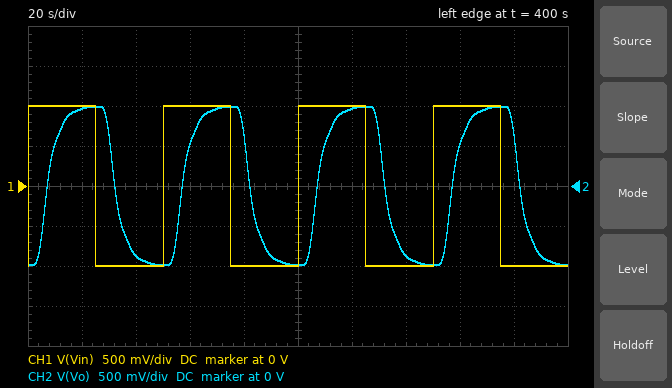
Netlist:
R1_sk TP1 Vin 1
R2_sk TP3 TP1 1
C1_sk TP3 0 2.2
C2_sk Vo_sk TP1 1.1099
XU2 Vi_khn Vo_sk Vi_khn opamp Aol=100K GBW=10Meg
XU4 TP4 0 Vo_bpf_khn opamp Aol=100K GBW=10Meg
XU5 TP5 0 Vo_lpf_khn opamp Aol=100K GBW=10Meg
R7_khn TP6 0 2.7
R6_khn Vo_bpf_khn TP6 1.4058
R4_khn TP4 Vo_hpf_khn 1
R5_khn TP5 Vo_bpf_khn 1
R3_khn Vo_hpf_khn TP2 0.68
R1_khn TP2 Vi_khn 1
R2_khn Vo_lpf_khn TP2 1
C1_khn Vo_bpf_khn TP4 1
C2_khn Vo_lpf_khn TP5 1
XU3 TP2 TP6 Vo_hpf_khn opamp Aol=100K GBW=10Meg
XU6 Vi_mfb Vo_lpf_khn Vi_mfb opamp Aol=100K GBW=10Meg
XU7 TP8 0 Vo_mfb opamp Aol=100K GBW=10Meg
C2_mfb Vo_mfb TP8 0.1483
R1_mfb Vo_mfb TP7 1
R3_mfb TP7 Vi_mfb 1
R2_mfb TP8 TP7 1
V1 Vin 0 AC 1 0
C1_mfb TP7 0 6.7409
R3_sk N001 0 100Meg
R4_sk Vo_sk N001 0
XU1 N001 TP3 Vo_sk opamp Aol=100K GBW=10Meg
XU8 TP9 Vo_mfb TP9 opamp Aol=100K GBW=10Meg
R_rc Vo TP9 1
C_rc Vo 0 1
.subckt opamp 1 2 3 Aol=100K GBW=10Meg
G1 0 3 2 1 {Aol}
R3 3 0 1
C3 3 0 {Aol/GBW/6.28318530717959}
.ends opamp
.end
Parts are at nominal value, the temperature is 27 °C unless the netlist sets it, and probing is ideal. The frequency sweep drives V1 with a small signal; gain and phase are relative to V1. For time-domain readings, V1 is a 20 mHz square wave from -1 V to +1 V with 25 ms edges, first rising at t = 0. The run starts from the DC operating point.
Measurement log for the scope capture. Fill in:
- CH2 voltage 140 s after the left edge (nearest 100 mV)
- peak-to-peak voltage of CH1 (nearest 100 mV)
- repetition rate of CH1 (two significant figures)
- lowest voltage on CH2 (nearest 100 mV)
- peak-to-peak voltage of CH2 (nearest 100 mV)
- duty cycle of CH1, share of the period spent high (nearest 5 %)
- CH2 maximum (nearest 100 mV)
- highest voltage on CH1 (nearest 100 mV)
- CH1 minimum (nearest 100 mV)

-900 mV
2.0 V
20 mHz
-1.0 V
2.0 V
50 %
1.0 V
1.0 V
-1.0 V
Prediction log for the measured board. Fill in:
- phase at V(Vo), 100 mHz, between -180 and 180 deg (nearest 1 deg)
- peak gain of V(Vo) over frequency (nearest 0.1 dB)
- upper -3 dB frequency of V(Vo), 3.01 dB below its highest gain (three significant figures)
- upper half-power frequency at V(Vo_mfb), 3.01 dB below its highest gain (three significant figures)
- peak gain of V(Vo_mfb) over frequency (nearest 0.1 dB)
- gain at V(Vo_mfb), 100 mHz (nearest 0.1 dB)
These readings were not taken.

140 deg
0 dB
38.1 mHz
40.2 mHz
0 dB
-8.8 dB
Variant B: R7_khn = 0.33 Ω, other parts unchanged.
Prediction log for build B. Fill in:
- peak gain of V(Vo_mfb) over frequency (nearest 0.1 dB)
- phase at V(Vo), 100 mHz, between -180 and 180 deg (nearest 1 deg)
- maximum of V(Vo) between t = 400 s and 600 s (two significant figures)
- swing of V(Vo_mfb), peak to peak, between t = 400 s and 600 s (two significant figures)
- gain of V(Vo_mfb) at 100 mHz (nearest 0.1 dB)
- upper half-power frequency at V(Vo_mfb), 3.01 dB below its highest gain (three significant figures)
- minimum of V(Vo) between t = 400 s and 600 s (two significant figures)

0.4 dB
169 deg
1.0 V
2.1 V
-0.7 dB
152 mHz
-1.0 V
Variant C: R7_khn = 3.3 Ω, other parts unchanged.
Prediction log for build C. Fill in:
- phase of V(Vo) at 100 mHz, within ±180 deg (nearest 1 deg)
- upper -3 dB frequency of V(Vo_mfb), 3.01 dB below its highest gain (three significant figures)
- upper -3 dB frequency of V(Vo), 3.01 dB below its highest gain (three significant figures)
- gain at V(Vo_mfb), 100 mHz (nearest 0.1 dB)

139 deg
38.8 mHz
36.9 mHz
-9.3 dB
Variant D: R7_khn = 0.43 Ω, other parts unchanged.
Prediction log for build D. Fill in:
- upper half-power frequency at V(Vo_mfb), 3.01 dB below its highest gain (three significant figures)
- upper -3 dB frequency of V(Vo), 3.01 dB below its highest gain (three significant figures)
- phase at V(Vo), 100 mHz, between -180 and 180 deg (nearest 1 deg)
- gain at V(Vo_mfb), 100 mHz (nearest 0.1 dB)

145 mHz
60.3 mHz
163 deg
-1.7 dB
